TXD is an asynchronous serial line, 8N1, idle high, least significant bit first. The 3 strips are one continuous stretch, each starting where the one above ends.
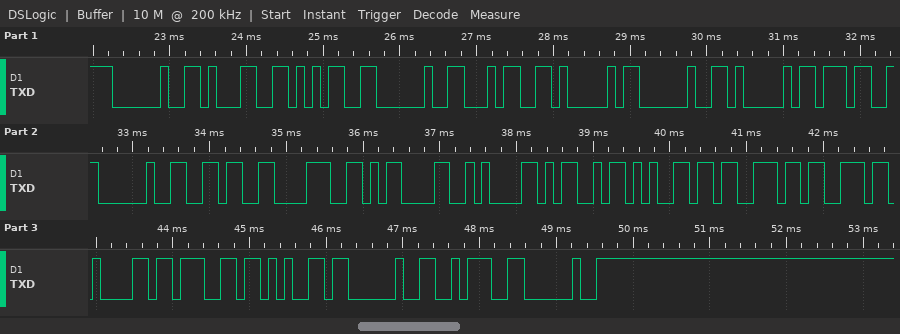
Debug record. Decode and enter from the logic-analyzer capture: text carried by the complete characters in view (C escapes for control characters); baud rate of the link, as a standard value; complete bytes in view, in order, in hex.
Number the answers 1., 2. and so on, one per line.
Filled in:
1. " 15 4A A7 68\r\nMessage : "
2. 9600 baud
3. 20 31 35 20 34 41 20 41 37 20 36 38 0D 0A 4D 65 73 73 61 67 65 20 3A 20
